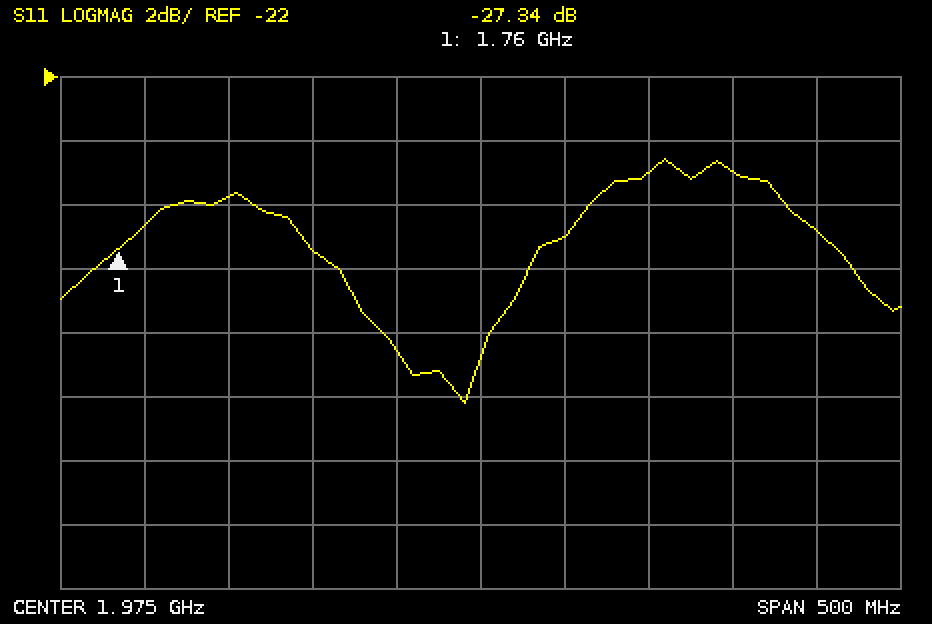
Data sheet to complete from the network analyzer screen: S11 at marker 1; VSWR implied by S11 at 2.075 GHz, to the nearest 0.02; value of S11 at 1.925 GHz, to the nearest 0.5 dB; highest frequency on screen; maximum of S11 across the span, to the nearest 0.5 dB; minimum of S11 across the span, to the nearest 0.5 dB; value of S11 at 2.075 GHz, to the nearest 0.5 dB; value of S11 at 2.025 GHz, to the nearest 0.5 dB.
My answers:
-27.34 dB
1.12
-30.5 dB
2.225 GHz
-24.5 dB
-32.0 dB
-25.0 dB
-27.0 dB
